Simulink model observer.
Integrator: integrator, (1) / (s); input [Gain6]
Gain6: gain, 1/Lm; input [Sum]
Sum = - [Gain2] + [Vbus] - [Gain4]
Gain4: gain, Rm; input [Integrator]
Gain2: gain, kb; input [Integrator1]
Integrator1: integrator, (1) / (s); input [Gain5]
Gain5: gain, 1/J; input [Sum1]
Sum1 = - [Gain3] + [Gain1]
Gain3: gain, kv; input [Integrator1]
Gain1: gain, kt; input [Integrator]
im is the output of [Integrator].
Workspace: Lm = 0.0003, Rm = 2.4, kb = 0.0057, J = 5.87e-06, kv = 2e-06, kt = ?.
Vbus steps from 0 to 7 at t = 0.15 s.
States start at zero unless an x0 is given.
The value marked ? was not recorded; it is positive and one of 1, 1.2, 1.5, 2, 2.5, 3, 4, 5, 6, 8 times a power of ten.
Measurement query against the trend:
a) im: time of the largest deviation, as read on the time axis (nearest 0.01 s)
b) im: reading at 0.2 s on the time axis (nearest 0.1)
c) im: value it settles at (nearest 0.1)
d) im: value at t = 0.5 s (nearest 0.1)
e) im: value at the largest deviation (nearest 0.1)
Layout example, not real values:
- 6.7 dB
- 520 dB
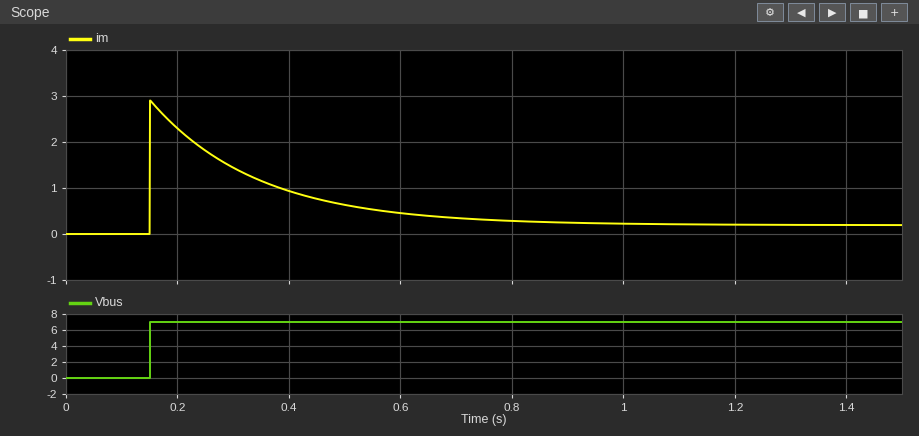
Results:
- 0.15 s
- 2.3
- 0.2
- 0.6
- 2.9
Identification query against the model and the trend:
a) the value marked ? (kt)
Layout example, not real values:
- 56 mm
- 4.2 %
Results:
- 0.012
